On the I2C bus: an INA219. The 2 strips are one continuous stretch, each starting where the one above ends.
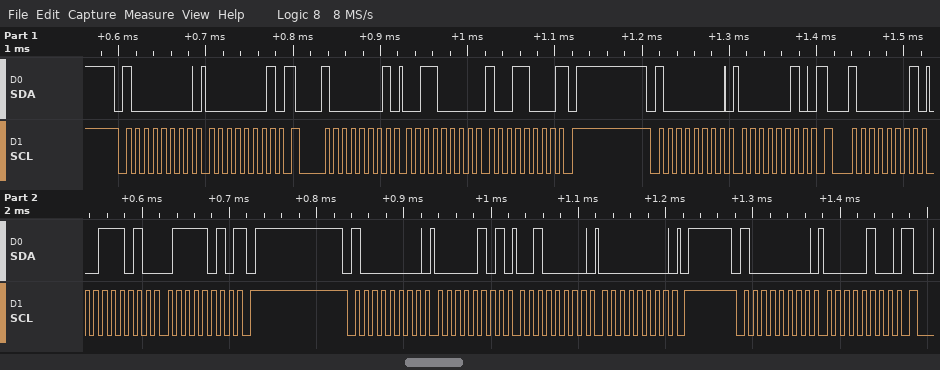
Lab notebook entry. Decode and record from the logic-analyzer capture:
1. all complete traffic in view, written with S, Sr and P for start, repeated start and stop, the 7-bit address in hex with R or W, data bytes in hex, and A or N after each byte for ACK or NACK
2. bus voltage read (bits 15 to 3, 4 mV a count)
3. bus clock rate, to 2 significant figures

S 40W A 01 A Sr 40R A 30 A 98 N P S 40W A 02 A Sr 40R A 3A A 7A N P S 40W A 05 A 20 A 00 A P S 40W A 04 A
7.484 V
100 kHz
